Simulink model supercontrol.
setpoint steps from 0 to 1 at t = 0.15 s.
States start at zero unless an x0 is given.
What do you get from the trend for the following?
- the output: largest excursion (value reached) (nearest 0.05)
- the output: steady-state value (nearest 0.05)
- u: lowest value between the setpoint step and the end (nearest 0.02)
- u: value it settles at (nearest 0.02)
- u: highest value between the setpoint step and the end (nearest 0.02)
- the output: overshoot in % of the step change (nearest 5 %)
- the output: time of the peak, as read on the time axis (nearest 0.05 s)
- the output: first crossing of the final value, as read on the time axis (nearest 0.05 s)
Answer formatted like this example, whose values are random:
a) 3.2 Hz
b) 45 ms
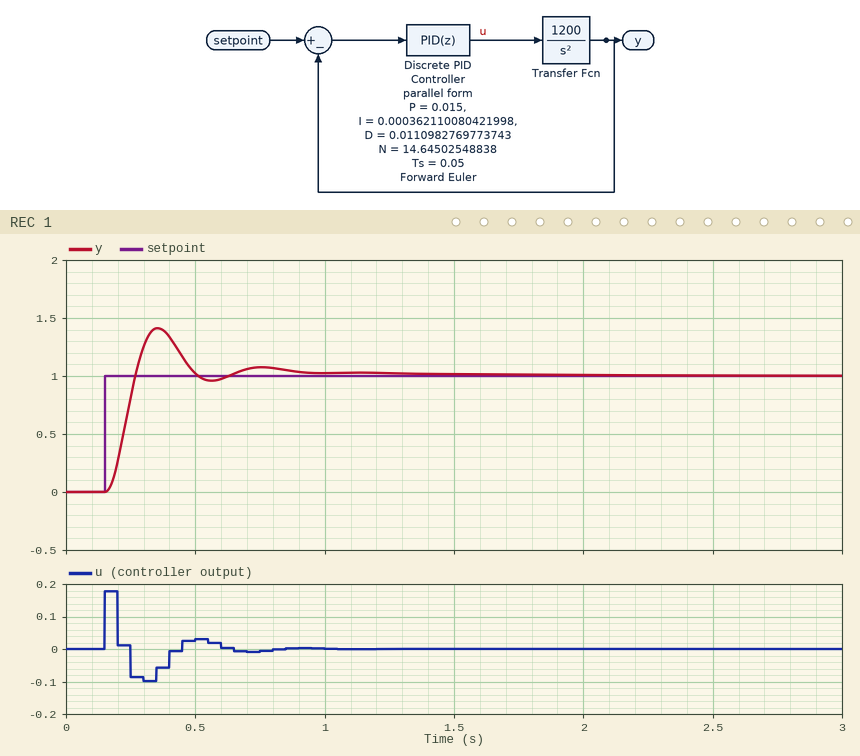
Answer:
a) 1.40
b) 1.00
c) -0.10
d) 0.00
e) 0.18
f) 40 %
g) 0.35 s
h) 0.25 s
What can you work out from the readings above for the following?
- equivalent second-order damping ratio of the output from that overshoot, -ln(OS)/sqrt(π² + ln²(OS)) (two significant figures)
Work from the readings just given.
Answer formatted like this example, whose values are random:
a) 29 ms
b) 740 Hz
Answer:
a) 0.28
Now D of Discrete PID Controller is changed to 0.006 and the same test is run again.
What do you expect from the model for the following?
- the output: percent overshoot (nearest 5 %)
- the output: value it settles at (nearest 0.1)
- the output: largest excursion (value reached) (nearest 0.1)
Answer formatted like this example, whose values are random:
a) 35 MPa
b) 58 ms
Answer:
a) 35 %
b) 1.0
c) 1.3
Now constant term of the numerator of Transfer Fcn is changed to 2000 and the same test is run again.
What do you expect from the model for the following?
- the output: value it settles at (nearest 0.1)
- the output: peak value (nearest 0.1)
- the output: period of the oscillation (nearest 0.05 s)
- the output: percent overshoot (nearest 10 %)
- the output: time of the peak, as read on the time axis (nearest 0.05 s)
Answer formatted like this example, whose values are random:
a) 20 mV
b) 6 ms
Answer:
a) 1.0
b) 1.7
c) 0.30 s
d) 70 %
e) 0.30 s
